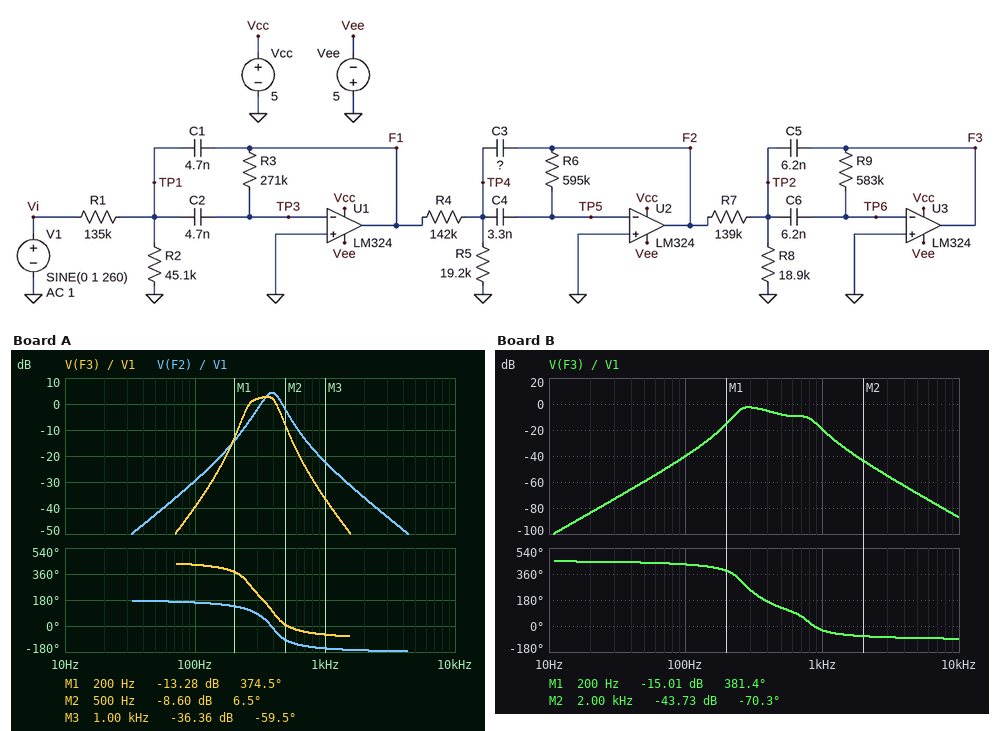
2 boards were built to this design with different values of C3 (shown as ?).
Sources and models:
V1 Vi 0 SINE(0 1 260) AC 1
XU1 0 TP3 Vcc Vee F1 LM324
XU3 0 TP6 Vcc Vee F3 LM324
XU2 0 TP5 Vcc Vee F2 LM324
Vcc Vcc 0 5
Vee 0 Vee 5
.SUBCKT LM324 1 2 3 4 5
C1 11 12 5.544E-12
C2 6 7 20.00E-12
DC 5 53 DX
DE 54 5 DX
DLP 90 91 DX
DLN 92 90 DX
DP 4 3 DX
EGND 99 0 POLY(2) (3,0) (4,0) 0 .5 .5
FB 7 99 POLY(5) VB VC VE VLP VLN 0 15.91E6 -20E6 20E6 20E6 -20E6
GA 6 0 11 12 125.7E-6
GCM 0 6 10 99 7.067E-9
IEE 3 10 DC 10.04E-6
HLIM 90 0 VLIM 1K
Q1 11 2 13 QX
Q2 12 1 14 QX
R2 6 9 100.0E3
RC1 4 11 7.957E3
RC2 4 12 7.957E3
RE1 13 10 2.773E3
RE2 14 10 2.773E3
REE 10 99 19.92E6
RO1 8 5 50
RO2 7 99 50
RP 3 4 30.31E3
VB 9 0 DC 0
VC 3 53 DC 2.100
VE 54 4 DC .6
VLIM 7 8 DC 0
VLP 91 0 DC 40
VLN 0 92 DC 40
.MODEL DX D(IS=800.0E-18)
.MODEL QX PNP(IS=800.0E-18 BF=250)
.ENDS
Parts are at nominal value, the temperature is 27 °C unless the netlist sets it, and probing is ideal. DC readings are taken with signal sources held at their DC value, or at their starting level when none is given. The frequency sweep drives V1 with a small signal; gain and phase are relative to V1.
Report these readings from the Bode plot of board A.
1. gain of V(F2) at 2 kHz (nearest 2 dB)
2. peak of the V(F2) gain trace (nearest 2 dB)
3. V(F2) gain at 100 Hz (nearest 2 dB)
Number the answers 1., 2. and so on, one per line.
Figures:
1. -36 dB
2. 4 dB
3. -30 dB
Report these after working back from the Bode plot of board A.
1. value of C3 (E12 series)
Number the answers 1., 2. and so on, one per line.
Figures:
1. 4.7 nF
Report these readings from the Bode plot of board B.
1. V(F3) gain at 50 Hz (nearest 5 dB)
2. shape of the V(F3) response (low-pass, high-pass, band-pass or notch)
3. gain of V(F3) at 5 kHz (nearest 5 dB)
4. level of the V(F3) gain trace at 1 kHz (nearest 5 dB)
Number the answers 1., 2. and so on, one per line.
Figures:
1. -60 dB
2. band-pass
3. -70 dB
4. -20 dB
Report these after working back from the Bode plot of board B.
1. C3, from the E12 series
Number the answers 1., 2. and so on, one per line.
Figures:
1. 1.2 nF
